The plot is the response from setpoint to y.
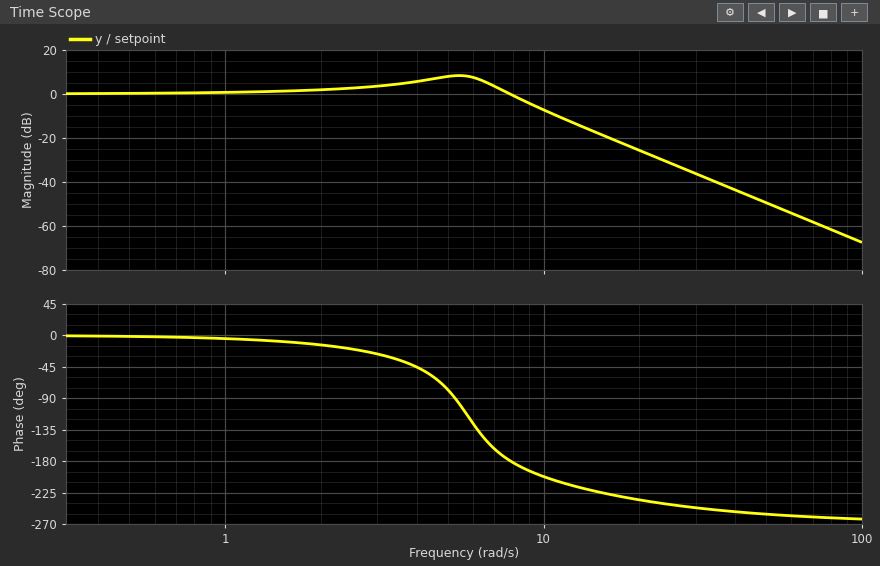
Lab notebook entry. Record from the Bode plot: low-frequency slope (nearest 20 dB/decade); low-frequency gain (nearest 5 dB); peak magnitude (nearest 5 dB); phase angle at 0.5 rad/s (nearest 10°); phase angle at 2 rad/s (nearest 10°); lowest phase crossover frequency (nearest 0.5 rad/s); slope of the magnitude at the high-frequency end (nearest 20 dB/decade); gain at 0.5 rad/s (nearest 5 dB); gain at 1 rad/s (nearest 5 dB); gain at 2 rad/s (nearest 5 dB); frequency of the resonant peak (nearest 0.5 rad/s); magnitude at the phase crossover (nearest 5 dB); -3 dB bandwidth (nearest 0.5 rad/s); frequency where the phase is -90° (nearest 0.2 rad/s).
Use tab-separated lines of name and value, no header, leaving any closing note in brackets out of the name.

low-frequency slope	0 dB/decade
low-frequency gain	0 dB
peak magnitude	10 dB
phase angle at 0.5 rad/s	0°
phase angle at 2 rad/s	-10°
lowest phase crossover frequency	8.0 rad/s
slope of the magnitude at the high-frequency end	-60 dB/decade
gain at 0.5 rad/s	0 dB
gain at 1 rad/s	0 dB
gain at 2 rad/s	0 dB
frequency of the resonant peak	5.5 rad/s
magnitude at the phase crossover	0 dB
-3 dB bandwidth	8.5 rad/s
frequency where the phase is -90°	5.2 rad/s
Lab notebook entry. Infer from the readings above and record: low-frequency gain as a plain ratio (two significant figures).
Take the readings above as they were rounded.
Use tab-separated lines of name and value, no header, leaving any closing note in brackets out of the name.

low-frequency gain as a plain ratio	1.0
